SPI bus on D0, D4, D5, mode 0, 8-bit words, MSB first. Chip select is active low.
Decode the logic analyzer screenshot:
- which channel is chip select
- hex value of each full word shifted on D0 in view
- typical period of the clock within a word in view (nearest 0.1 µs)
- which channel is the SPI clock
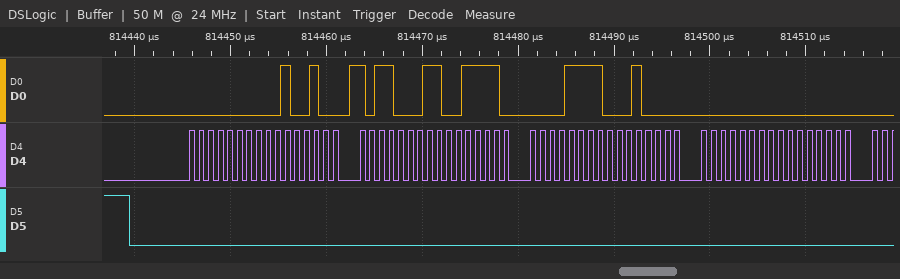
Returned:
D5
00, 24, B1, 9E, 0F, 10, 00, 00
1 µs
D4
